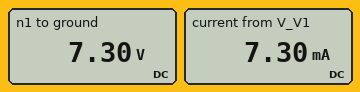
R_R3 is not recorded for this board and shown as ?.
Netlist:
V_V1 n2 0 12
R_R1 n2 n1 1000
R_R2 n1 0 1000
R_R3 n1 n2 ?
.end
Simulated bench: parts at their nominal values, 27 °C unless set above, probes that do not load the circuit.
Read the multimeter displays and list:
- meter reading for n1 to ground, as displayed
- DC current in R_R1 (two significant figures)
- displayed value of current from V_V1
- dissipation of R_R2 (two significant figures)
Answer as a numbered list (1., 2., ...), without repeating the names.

1. 7.30 V
2. 4.7 mA
3. 7.30 mA
4. 53 mW
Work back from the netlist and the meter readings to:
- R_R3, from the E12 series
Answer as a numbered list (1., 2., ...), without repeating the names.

1. 1.8 kΩ
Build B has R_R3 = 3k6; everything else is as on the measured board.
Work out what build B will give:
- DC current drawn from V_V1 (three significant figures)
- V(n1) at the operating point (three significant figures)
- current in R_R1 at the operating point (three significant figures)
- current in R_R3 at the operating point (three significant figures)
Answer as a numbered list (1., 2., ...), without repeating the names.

1. 6.73 mA
2. 6.73 V
3. 5.27 mA
4. 1.46 mA
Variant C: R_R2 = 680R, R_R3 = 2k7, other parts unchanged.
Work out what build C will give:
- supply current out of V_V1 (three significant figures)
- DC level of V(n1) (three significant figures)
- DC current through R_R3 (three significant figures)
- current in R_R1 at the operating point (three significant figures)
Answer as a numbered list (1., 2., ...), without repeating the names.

1. 8.51 mA
2. 5.79 V
3. 2.30 mA
4. 6.21 mA
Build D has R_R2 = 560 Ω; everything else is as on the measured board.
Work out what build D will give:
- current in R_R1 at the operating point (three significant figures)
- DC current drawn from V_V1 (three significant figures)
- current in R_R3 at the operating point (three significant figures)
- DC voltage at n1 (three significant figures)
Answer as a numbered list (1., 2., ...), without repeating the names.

1. 6.41 mA
2. 9.98 mA
3. 3.56 mA
4. 5.59 V
